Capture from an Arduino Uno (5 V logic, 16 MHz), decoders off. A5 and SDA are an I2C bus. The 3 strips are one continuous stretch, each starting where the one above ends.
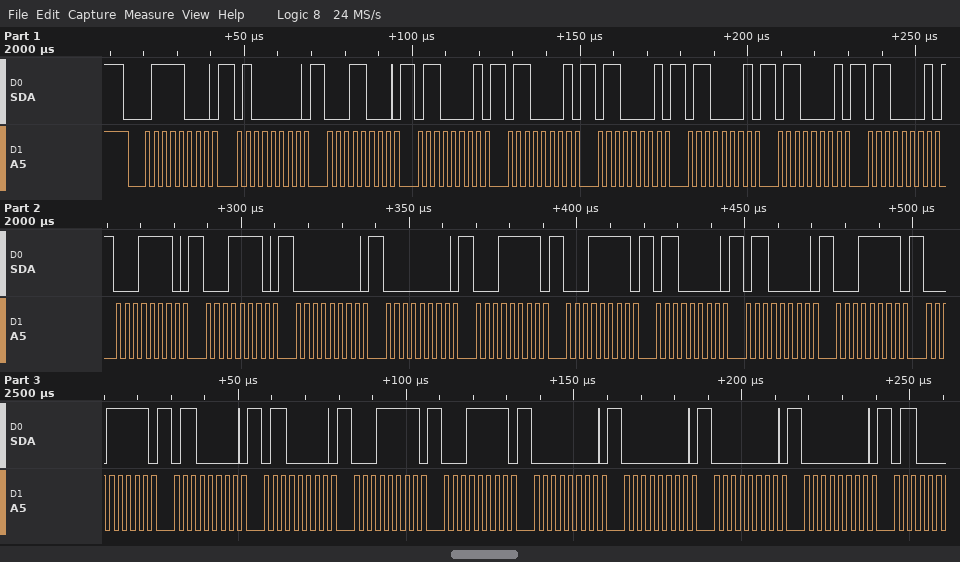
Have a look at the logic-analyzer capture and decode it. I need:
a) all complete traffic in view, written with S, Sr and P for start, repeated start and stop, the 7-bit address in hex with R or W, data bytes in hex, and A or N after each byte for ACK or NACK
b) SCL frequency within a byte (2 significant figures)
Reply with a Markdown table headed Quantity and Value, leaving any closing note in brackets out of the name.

| Quantity | Value |
|---|---|
| all complete traffic in view, written with S, Sr and P for start, repeated start and stop, the 7-bit address in hex with R or W, data bytes in hex, and A or N after each byte for ACK or NACK | S 3CW A 40 A 18 A 61 A 61 A 61 A 61 A 61 A 61 A 1E A 1E A 00 A 00 A 1F A 1F A 60 A 60 A 1F A 1F A 60 A 60 A 1F A 1F A 00 A 00 A 00 A 00 A |
| SCL frequency within a byte | 400 kHz |
